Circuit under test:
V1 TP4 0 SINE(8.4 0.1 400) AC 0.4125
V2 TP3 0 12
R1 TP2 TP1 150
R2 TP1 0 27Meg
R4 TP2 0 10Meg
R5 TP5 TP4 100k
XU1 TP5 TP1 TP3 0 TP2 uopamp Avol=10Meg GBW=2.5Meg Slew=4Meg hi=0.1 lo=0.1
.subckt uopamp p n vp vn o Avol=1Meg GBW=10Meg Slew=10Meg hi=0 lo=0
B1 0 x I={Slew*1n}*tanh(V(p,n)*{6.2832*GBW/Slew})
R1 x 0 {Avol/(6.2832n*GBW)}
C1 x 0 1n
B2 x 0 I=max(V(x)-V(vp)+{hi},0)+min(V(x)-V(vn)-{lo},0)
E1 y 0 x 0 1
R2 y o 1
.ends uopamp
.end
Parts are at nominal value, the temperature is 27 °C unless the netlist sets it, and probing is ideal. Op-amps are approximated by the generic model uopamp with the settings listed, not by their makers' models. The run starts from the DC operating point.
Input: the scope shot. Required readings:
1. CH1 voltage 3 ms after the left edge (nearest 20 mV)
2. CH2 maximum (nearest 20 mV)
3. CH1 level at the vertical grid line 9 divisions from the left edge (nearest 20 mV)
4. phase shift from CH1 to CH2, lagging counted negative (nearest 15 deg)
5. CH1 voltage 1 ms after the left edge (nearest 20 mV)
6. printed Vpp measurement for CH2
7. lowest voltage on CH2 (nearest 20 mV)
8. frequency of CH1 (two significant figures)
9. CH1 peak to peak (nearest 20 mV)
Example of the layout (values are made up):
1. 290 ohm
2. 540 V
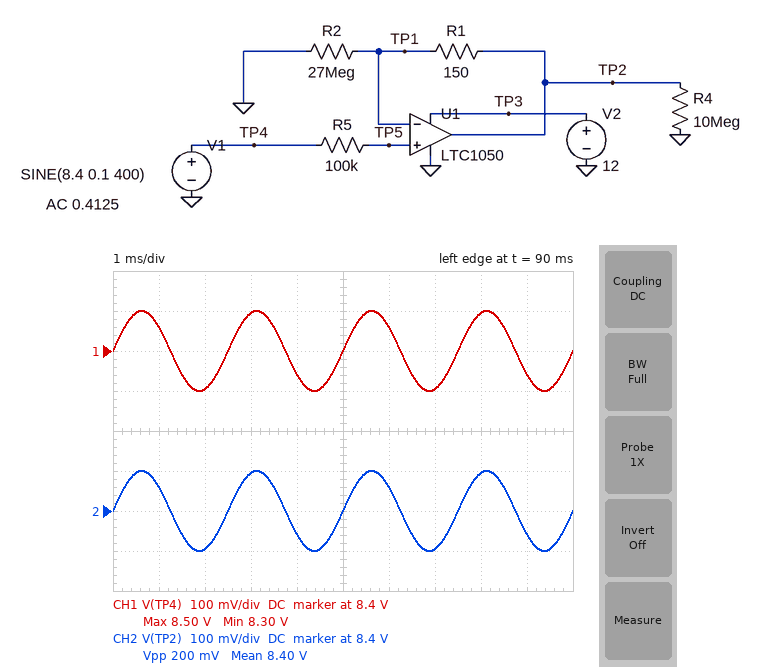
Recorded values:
1. 8.50 V
2. 8.50 V
3. 8.34 V
4. 0 deg
5. 8.46 V
6. 200 mV
7. 8.30 V
8. 400 Hz
9. 200 mV
